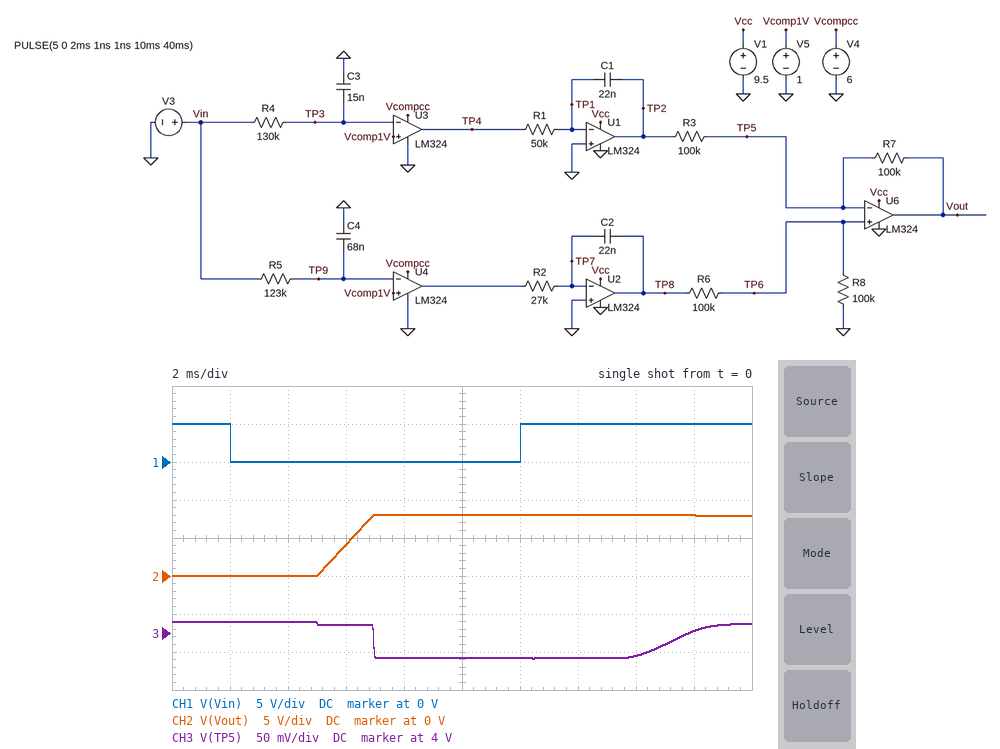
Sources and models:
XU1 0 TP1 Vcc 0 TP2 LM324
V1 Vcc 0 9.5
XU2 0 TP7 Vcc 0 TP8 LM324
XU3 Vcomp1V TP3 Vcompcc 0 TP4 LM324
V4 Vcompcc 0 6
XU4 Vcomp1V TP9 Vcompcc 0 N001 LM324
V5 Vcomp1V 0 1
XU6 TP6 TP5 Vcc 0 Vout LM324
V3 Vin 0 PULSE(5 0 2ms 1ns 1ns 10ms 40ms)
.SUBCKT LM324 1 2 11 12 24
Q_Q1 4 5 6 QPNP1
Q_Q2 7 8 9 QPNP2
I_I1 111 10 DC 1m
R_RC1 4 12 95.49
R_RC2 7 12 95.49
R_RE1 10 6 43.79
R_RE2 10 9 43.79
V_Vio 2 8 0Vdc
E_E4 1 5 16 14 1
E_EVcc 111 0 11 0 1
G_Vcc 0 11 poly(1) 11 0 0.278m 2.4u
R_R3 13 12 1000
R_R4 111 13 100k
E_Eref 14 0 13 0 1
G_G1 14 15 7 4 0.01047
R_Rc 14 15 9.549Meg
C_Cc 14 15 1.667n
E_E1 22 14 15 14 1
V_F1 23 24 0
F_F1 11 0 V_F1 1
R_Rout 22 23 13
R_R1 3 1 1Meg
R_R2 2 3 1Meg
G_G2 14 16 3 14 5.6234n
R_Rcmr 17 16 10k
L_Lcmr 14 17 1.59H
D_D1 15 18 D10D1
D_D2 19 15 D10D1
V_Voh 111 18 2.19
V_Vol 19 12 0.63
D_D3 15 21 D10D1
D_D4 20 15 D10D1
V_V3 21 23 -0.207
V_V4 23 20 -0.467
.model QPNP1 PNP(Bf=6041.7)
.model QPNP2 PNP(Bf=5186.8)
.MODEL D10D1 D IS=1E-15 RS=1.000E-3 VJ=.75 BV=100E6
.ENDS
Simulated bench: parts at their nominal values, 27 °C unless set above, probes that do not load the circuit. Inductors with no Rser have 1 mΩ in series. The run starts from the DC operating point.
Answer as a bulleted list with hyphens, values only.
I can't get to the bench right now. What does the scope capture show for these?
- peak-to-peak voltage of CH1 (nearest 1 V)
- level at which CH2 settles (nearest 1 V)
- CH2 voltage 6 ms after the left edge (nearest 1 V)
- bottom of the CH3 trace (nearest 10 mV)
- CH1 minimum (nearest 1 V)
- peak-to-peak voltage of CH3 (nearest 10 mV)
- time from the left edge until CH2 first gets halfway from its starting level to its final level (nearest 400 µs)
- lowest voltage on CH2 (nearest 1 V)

- 5 V
- 8 V
- 4 V
- 3.97 V
- 0 V
- 50 mV
- 6.0 ms
- 0 V
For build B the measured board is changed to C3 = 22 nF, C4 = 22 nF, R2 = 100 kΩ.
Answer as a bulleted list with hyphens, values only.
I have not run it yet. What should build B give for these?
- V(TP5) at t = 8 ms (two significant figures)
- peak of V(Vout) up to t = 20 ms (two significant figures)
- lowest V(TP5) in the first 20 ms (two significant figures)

- 2.1 V
- 3.6 V
- -35 mV
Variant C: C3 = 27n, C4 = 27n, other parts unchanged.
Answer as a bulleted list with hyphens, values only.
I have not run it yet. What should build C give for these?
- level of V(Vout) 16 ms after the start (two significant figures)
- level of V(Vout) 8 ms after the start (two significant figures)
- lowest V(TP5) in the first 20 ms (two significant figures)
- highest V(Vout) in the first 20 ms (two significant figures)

- 160 mV
- -84 mV
- -36 mV
- 470 mV
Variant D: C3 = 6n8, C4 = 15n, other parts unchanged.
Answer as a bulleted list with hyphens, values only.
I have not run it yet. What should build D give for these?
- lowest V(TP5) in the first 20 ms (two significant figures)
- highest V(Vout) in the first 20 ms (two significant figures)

- -36 mV
- 6.0 V
